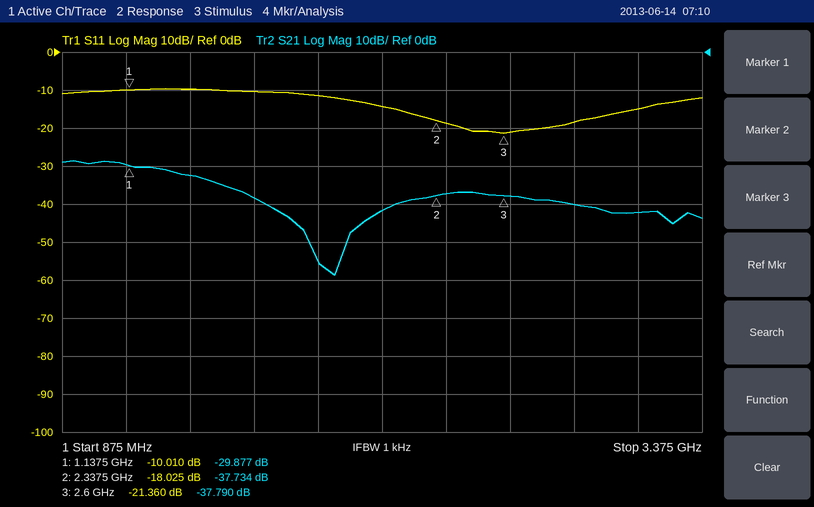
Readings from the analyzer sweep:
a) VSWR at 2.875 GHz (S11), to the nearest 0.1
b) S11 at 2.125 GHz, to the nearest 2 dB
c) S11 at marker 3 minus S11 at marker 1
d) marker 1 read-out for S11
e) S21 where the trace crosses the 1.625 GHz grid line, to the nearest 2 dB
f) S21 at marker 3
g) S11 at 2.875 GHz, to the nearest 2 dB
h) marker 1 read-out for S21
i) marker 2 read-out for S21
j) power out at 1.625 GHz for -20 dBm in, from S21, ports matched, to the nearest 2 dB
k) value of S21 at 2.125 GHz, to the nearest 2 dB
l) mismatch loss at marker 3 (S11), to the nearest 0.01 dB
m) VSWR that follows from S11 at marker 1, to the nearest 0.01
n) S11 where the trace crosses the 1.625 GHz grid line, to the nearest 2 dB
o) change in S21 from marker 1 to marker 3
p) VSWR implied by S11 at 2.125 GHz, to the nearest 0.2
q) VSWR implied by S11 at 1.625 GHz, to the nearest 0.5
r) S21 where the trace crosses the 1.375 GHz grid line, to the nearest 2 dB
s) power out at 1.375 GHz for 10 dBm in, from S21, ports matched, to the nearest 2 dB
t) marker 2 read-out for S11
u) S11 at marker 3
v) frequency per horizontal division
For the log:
1.3
-14 dB
-11.350 dB
-10.010 dB
-38 dB
-37.790 dB
-18 dB
-29.877 dB
-37.734 dB
-58 dBm
-42 dB
0.03 dB
1.92
-10 dB
-7.913 dB
1.4
2.0
-32 dB
-22 dBm
-18.025 dB
-21.360 dB
250 MHz
